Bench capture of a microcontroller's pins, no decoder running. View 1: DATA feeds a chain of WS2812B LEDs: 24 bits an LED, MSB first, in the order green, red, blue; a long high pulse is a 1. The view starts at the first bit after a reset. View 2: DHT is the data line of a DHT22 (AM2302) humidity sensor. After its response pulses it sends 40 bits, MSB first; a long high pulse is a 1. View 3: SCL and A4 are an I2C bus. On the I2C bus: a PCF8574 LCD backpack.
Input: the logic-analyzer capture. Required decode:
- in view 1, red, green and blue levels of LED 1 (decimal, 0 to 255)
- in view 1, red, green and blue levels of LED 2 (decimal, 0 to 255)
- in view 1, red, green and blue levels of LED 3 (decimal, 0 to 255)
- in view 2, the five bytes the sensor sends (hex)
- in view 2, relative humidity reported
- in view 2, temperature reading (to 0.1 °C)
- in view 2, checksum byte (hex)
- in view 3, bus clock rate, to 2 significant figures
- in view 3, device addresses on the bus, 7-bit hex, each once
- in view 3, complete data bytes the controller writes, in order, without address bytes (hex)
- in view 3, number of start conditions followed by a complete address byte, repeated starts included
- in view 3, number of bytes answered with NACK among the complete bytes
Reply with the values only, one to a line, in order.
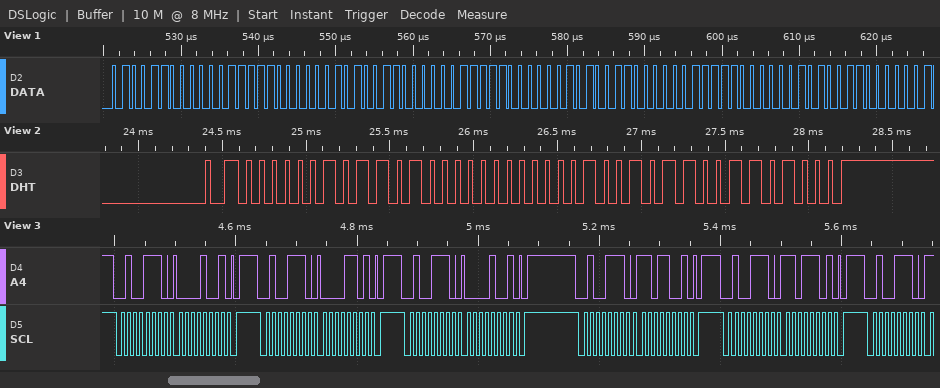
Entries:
15, 76, 129
15, 76, 129
15, 76, 129
02 D0 00 96 68
72.0 %
15.0 °C
0x68
100 kHz
0x27
09 0D 09 D9 DD
6
0
